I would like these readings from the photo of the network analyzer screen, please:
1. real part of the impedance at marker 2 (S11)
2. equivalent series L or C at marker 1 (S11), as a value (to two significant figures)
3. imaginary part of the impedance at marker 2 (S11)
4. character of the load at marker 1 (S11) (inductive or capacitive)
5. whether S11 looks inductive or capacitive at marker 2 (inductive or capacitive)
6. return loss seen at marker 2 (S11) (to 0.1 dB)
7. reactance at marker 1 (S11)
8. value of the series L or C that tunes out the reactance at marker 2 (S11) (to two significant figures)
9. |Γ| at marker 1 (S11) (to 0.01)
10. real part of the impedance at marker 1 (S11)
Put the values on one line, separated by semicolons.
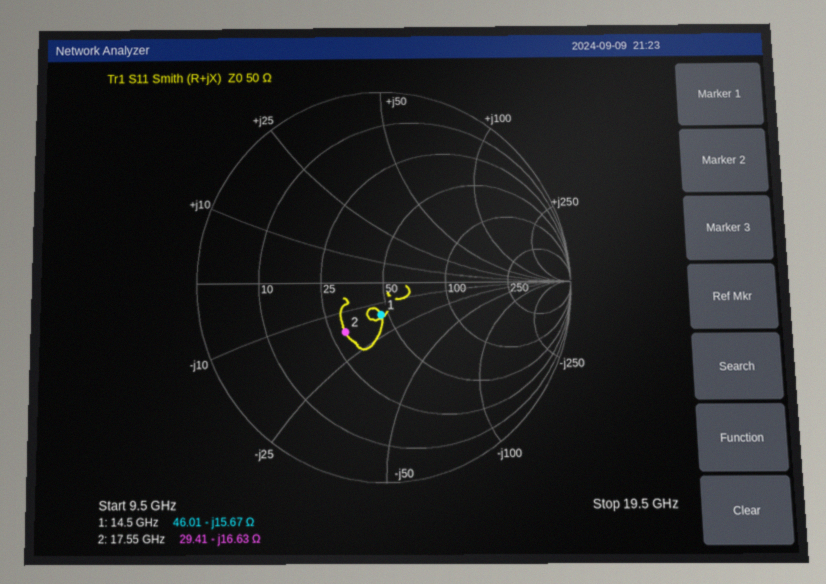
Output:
29.41 Ω; 700 fF; -16.63 Ω; capacitive; capacitive; 9.7 dB; -15.67 Ω; 150 pH; 0.17; 46.01 Ω
